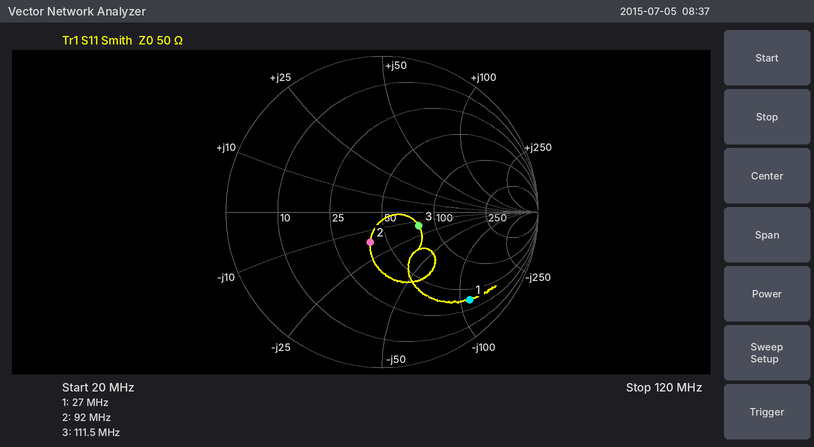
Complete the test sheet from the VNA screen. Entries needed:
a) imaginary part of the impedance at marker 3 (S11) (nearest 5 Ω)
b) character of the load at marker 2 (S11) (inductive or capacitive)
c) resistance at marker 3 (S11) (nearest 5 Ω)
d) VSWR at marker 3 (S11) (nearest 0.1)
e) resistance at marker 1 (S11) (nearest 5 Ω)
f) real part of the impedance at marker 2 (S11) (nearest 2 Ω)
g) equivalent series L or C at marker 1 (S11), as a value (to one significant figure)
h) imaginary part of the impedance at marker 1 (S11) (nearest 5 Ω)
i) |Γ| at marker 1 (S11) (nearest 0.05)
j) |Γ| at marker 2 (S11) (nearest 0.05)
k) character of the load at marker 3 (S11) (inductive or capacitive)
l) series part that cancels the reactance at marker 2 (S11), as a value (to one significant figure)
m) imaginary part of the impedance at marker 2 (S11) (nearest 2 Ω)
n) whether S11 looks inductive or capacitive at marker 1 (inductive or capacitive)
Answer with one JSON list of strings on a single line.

["-15 Ω", "capacitive", "80 Ω", "1.7", "35 Ω", "40 Ω", "50 pF", "-110 Ω", "0.80", "0.20", "capacitive", "30 nH", "-16 Ω", "capacitive"]
